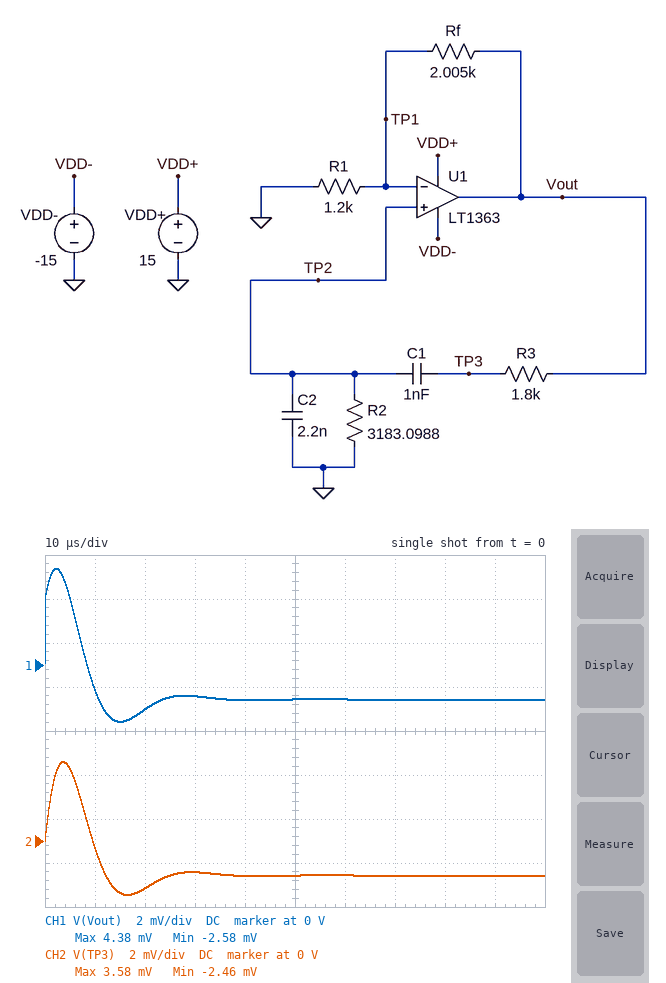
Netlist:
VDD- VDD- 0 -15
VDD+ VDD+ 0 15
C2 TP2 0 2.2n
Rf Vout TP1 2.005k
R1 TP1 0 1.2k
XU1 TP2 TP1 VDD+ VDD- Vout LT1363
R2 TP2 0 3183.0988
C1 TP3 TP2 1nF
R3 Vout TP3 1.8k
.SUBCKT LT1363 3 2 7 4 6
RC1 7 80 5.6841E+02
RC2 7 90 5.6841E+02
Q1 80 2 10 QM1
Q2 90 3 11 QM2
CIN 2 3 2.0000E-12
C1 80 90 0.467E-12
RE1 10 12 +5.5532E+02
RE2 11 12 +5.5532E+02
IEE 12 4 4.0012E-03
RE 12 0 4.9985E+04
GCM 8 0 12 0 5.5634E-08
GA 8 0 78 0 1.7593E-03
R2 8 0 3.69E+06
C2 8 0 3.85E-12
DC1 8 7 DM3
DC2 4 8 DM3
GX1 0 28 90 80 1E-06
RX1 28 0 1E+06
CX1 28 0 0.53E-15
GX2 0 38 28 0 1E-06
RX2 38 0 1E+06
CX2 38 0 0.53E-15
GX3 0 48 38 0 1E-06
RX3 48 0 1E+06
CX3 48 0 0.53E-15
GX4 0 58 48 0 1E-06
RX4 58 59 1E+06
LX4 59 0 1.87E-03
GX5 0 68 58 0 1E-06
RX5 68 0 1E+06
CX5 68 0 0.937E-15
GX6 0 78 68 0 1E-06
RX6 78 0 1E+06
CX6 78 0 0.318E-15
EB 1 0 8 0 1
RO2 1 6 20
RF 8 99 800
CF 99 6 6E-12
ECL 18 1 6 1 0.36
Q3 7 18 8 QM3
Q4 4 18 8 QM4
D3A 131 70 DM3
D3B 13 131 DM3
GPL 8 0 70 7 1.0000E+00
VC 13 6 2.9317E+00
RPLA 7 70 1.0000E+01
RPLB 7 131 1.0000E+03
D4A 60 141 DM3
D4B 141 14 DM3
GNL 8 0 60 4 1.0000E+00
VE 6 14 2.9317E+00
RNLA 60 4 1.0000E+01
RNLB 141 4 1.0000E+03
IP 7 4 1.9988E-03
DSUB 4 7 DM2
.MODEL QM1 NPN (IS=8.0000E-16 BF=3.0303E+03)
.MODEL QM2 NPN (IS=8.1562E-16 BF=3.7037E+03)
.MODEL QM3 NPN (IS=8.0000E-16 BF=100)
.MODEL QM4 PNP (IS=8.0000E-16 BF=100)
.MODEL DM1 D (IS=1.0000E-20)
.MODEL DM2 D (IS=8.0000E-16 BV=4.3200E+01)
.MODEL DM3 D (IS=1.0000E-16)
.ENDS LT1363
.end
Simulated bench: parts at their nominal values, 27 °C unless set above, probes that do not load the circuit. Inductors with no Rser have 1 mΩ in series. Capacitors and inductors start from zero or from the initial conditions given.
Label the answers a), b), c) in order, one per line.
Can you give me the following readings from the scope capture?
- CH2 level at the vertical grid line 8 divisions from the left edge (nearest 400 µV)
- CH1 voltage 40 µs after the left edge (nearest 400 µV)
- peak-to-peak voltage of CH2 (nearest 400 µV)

a) -1.6 mV
b) -1.6 mV
c) 6.0 mV
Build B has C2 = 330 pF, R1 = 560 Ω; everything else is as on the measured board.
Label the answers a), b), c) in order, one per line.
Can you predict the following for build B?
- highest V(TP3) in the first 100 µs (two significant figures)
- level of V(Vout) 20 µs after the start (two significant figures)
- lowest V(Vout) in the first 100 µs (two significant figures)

a) 12 V
b) 14 V
c) -14 V
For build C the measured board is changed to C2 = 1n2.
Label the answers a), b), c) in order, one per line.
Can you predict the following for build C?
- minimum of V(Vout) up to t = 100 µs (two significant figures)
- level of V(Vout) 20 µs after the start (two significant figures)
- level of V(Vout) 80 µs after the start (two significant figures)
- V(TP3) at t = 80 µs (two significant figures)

a) -8.0 mV
b) 3.4 mV
c) -2.2 mV
d) -2.5 mV
